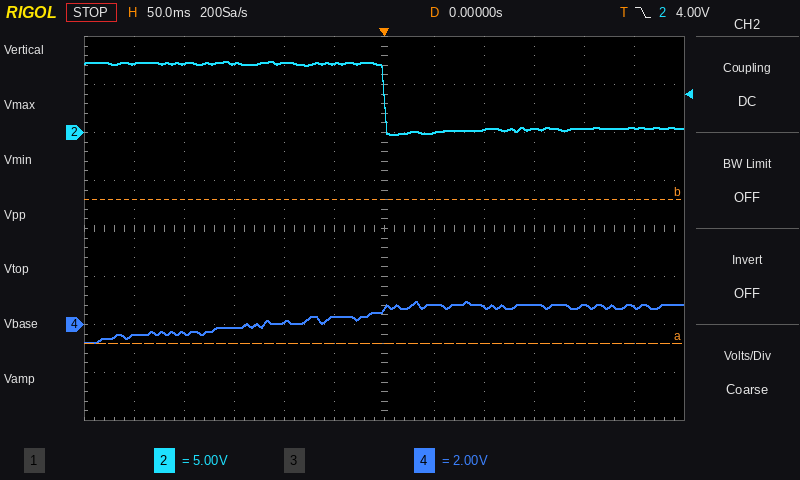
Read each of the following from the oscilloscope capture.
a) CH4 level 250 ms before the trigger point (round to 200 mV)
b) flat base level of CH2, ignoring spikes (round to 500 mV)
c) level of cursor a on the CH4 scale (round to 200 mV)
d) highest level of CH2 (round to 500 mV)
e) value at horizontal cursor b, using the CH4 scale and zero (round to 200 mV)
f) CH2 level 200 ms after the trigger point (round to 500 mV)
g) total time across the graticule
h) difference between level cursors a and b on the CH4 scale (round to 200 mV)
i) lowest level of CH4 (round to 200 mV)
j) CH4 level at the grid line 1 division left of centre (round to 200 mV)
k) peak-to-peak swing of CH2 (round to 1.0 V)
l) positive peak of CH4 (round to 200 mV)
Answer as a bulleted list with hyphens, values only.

- -400 mV
- 500 mV
- -800 mV
- 7.5 V
- 5.2 V
- 500 mV
- 600 ms
- 6.0 V
- -800 mV
- 400 mV
- 8.0 V
- 1.0 V
